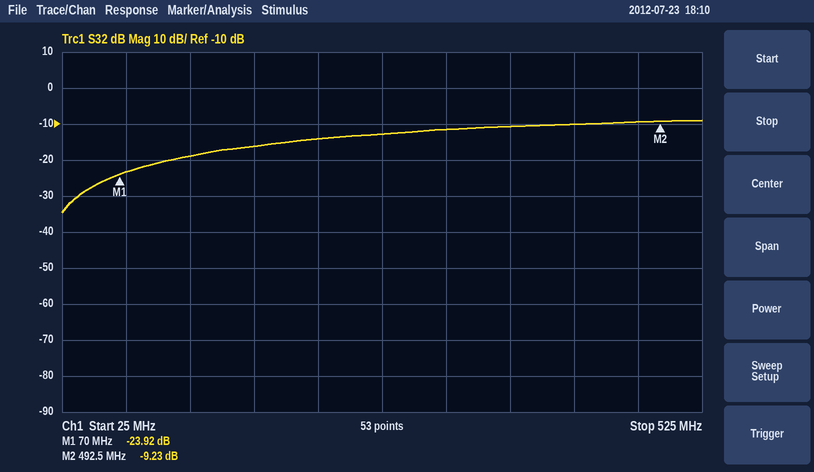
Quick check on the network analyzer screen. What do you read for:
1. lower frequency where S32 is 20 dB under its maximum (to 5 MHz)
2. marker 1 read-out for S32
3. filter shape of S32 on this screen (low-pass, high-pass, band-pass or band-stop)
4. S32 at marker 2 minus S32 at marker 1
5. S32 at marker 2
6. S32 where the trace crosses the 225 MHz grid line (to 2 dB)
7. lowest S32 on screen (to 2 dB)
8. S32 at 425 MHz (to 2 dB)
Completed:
40 MHz
-23.92 dB
high-pass
14.69 dB
-9.23 dB
-14 dB
-34 dB
-10 dB
